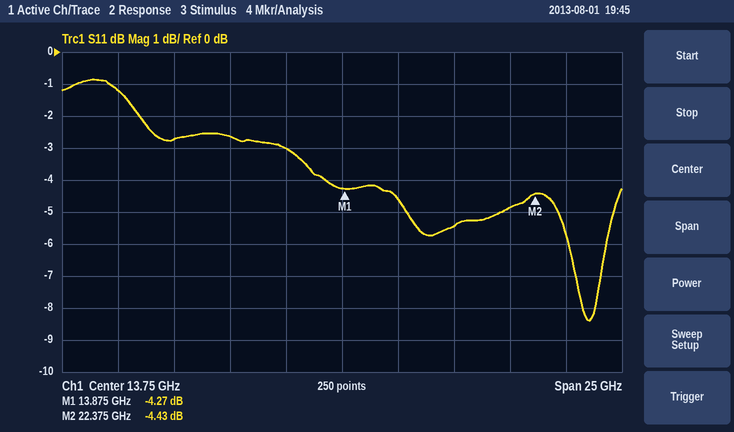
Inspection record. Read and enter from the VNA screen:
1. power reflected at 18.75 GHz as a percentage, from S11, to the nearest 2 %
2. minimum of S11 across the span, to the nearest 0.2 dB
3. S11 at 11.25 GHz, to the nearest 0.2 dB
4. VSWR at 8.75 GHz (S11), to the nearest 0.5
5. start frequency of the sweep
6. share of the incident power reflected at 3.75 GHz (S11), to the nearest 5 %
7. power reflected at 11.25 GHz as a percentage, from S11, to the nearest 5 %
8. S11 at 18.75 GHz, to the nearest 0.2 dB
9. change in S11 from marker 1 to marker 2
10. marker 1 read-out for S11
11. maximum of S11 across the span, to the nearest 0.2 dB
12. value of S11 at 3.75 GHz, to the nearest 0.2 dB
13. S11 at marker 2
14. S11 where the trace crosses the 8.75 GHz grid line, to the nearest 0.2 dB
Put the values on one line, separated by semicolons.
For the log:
28 %; -8.4 dB; -3.0 dB; 6.5; 1.25 GHz; 75 %; 50 %; -5.4 dB; -0.16 dB; -4.27 dB; -0.8 dB; -1.2 dB; -4.43 dB; -2.6 dB
